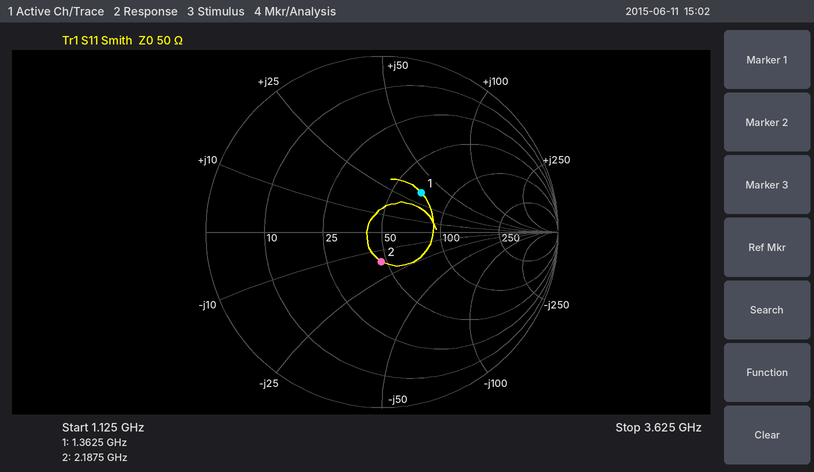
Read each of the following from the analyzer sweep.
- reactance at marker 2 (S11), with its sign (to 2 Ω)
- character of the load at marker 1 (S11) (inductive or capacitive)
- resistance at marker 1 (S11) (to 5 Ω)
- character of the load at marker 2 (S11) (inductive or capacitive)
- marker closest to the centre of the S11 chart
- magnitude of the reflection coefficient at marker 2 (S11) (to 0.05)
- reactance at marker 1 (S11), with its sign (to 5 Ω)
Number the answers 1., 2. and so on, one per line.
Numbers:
1. -16 Ω
2. inductive
3. 70 Ω
4. capacitive
5. marker 2
6. 0.15
7. +35 Ω
